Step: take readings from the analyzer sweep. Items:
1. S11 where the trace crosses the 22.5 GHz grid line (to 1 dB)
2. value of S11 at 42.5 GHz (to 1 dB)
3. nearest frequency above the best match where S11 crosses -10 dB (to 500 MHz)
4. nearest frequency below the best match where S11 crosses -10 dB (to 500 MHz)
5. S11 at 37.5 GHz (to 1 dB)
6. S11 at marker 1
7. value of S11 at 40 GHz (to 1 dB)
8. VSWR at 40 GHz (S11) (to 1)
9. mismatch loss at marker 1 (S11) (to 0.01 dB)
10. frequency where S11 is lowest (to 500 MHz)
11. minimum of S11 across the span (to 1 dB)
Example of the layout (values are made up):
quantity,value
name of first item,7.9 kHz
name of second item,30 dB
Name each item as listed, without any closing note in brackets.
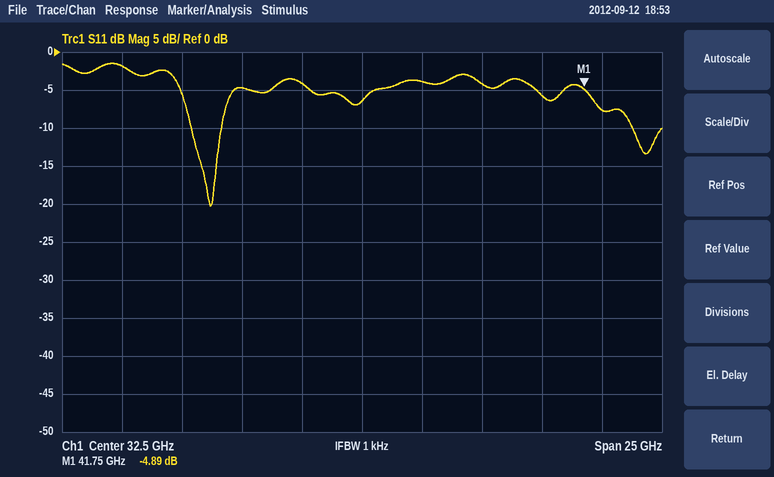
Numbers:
quantity,value
S11 where the trace crosses the 22.5 GHz grid line,-2 dB
value of S11 at 42.5 GHz,-8 dB
nearest frequency above the best match where S11 crosses -10 dB,26.5 GHz
nearest frequency below the best match where S11 crosses -10 dB,25.5 GHz
S11 at 37.5 GHz,-4 dB
S11 at marker 1,-4.89 dB
value of S11 at 40 GHz,-6 dB
VSWR at 40 GHz (S11),3
mismatch loss at marker 1 (S11),1.70 dB
frequency where S11 is lowest,26.0 GHz
minimum of S11 across the span,-20 dB
